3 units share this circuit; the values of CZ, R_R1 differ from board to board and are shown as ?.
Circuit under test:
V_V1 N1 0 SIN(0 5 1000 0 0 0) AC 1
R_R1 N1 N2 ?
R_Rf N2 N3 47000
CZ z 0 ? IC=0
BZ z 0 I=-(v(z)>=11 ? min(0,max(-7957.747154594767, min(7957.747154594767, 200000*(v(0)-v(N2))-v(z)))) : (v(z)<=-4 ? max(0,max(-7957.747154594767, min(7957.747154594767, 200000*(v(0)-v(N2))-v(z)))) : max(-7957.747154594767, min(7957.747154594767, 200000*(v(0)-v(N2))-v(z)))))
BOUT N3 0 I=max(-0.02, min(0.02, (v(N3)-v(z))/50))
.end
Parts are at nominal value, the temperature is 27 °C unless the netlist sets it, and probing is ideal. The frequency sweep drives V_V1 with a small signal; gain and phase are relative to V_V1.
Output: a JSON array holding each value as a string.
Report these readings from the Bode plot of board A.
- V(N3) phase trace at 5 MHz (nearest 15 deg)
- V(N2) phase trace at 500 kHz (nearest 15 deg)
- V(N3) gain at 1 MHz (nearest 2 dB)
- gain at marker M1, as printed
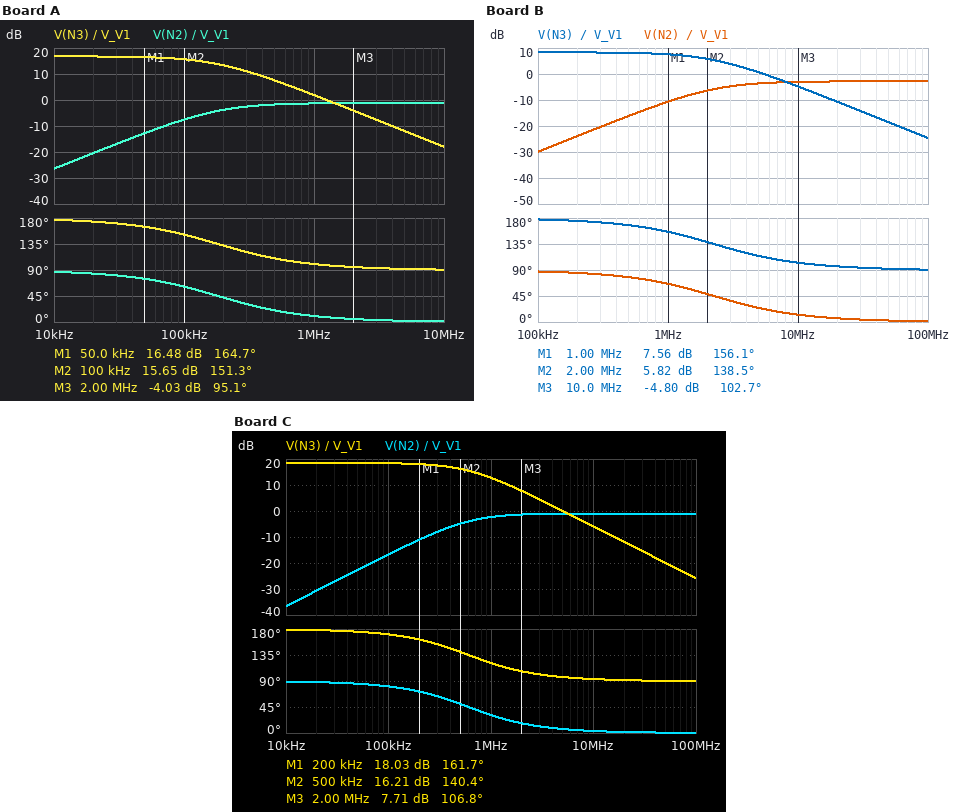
["90 deg", "15 deg", "2 dB", "16.48 dB"]
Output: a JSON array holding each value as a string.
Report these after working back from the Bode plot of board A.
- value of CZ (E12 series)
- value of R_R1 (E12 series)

["22 mF", "6.8 kΩ"]
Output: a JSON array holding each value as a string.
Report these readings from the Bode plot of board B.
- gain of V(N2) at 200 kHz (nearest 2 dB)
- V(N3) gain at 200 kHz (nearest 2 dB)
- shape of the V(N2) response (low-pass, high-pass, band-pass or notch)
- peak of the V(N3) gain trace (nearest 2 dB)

["-24 dB", "8 dB", "high-pass", "8 dB"]
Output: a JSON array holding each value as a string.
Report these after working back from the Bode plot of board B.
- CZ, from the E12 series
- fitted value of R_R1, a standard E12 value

["3.9 mF", "18 kΩ"]
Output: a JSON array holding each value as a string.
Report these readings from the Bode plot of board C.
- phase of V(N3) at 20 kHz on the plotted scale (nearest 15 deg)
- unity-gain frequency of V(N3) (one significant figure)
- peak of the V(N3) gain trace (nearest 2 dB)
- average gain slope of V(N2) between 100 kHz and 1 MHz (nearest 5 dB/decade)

["180 deg", "5 MHz", "18 dB", "15 dB/decade"]
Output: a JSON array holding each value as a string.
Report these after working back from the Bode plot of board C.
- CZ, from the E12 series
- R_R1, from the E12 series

["5.6 mF", "5.6 kΩ"]
